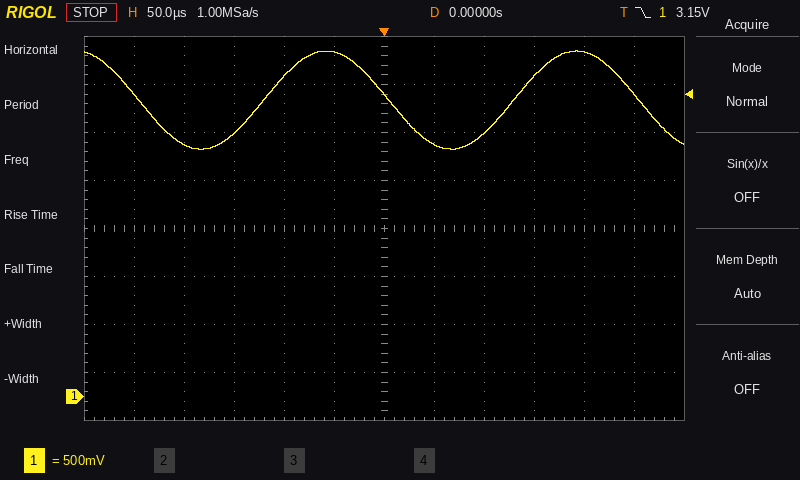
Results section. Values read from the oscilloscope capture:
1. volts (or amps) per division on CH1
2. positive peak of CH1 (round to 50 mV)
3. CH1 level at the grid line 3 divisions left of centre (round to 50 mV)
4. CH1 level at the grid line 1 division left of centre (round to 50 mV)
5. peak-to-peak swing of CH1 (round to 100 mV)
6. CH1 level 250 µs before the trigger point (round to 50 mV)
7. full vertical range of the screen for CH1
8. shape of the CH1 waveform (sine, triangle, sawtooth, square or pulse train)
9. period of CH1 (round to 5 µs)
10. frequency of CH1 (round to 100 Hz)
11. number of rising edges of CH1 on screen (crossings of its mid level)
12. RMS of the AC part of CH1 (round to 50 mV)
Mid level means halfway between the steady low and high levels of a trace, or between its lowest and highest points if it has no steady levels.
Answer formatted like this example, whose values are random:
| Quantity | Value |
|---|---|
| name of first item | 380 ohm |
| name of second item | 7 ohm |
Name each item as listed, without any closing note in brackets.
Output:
| Quantity | Value |
|---|---|
| volts (or amps) per division on CH1 | 500 mV |
| positive peak of CH1 | 3.60 V |
| CH1 level at the grid line 3 divisions left of centre | 2.75 V |
| CH1 level at the grid line 1 division left of centre | 3.60 V |
| peak-to-peak swing of CH1 | 1.00 V |
| CH1 level 250 µs before the trigger point | 3.15 V |
| full vertical range of the screen for CH1 | 4 V |
| shape of the CH1 waveform | sine |
| period of CH1 | 250 µs |
| frequency of CH1 | 4.0 kHz |
| number of rising edges of CH1 on screen | 2 |
| RMS of the AC part of CH1 | 350 mV |
